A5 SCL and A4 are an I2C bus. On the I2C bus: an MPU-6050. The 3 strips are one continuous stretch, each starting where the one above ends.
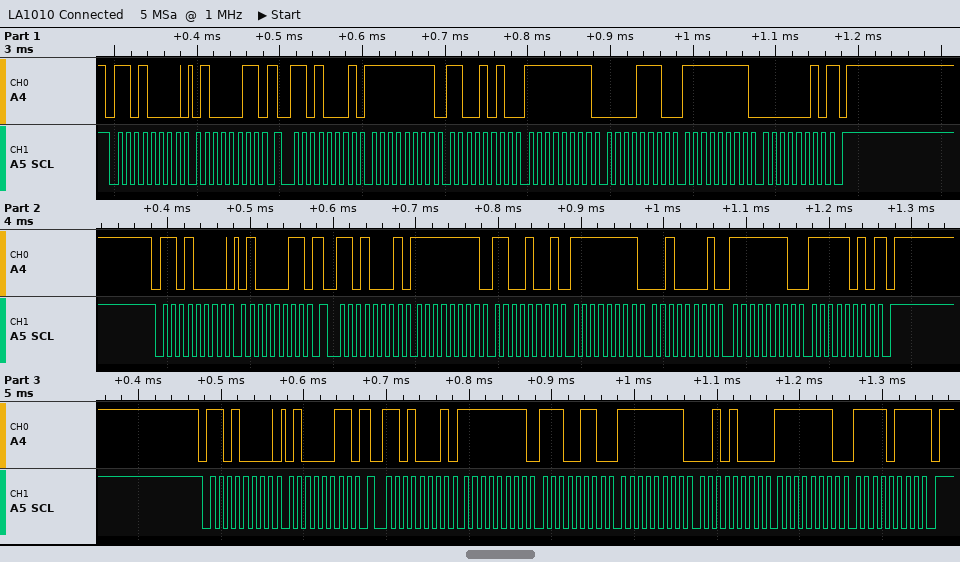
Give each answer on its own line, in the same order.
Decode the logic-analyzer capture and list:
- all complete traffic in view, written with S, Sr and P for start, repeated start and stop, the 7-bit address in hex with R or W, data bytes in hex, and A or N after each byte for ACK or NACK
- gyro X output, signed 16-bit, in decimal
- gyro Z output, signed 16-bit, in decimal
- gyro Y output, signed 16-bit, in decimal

S 68W A 43 A Sr 68R A FF A CA A FF A 0E A FF A 02 N P S 68W A 43 A Sr 68R A FF A C9 A FF A 21 A FE A FA N P S 68W A 43 A Sr 68R A FF A E6 A FF A 28 A FE A F7 N P
-54
-254
-242
